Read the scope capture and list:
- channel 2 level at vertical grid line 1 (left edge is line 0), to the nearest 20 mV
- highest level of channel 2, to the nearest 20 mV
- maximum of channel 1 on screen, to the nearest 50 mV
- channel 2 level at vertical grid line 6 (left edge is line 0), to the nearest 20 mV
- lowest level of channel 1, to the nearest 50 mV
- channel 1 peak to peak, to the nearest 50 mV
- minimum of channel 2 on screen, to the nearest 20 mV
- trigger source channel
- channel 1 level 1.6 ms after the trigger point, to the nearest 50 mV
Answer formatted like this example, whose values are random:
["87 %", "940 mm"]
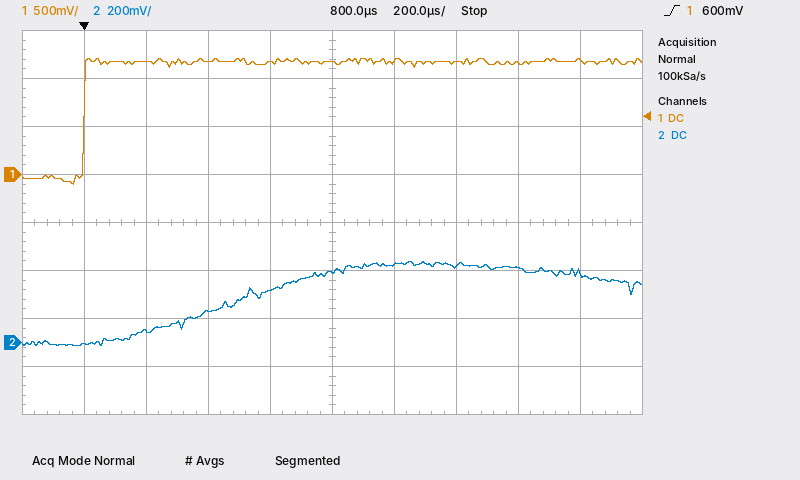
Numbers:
["0 mV", "340 mV", "1.20 V", "320 mV", "-100 mV", "1.30 V", "-20 mV", "channel 1", "1.20 V"]
